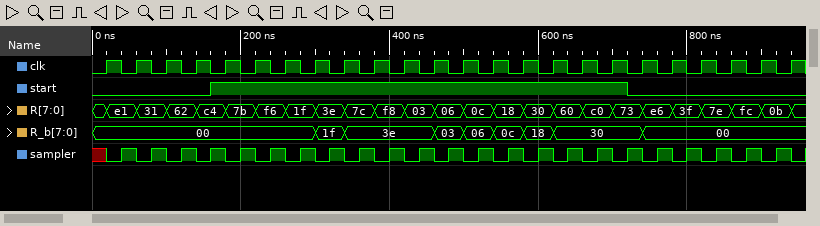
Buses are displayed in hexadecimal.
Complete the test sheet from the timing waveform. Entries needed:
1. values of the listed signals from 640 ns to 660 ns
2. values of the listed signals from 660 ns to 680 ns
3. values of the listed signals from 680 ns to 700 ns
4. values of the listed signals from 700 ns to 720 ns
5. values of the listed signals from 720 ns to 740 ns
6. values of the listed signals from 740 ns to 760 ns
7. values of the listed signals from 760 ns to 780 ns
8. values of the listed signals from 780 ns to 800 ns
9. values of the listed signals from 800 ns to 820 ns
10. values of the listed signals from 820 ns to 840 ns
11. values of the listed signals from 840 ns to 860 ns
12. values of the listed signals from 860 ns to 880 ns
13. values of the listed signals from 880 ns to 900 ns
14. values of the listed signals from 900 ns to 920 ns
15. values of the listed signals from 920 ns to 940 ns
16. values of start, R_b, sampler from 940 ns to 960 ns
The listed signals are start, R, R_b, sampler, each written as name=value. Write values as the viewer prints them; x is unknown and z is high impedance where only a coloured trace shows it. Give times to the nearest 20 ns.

start=1, R=60, R_b=30, sampler=1
start=1, R=c0, R_b=30, sampler=0
start=1, R=c0, R_b=30, sampler=1
start=1, R=73, R_b=30, sampler=0
start=0, R=73, R_b=30, sampler=1
start=0, R=e6, R_b=00, sampler=0
start=0, R=e6, R_b=00, sampler=1
start=0, R=3f, R_b=00, sampler=0
start=0, R=3f, R_b=00, sampler=1
start=0, R=7e, R_b=00, sampler=0
start=0, R=7e, R_b=00, sampler=1
start=0, R=fc, R_b=00, sampler=0
start=0, R=fc, R_b=00, sampler=1
start=0, R=0b, R_b=00, sampler=0
start=0, R=0b, R_b=00, sampler=1
start=0, R_b=00, sampler=0
